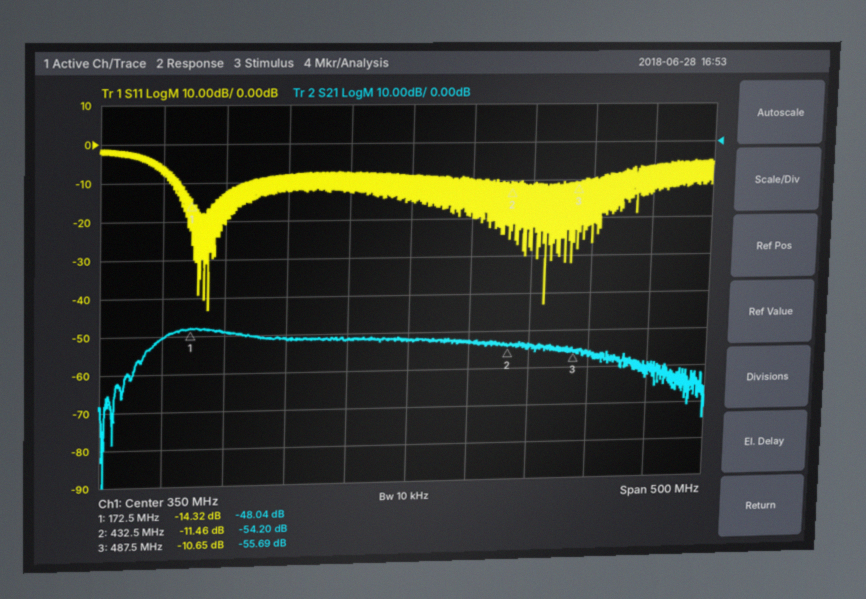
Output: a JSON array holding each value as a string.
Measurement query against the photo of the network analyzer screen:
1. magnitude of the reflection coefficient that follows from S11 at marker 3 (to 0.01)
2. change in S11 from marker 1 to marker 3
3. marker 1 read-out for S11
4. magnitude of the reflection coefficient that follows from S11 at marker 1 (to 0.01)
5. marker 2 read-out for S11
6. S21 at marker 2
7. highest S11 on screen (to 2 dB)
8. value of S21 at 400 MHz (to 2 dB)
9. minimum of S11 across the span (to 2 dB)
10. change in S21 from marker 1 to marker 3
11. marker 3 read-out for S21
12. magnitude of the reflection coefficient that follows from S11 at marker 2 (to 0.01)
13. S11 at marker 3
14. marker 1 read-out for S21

["0.29", "3.67 dB", "-14.32 dB", "0.19", "-11.46 dB", "-54.20 dB", "-2 dB", "-52 dB", "-44 dB", "-7.65 dB", "-55.69 dB", "0.27", "-10.65 dB", "-48.04 dB"]
